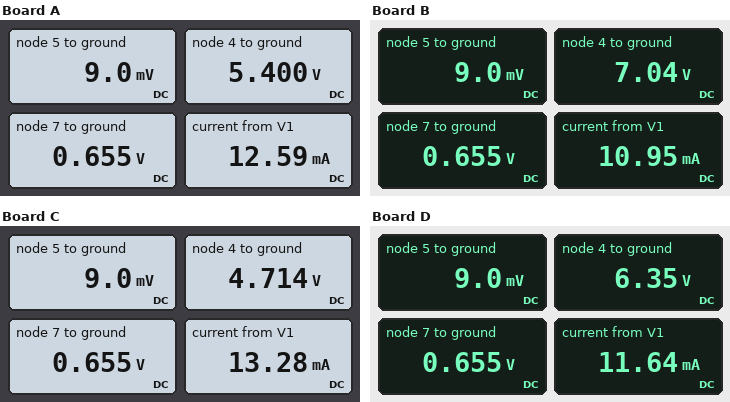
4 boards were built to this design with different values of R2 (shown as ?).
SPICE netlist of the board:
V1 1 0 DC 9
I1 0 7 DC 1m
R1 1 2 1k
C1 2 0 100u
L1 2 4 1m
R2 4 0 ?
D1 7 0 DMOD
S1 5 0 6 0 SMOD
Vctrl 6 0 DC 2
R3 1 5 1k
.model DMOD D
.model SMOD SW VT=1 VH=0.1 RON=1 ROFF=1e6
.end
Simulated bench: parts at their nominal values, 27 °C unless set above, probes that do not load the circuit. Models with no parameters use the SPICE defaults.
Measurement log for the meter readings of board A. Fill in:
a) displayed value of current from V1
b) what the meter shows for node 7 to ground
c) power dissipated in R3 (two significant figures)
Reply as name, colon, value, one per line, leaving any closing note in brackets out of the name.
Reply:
displayed value of current from V1: 12.59 mA
what the meter shows for node 7 to ground: 0.655 V
power dissipated in R3: 81 mW
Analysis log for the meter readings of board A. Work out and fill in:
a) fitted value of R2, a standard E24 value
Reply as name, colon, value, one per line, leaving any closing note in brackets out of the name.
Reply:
fitted value of R2, a standard E24 value: 1.5 kΩ
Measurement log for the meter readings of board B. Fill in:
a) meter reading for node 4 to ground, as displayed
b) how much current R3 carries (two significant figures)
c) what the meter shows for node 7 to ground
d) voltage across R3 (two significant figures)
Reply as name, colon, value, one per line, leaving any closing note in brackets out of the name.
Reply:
meter reading for node 4 to ground, as displayed: 7.04 V
how much current R3 carries: 9.0 mA
what the meter shows for node 7 to ground: 0.655 V
voltage across R3: 9.0 V
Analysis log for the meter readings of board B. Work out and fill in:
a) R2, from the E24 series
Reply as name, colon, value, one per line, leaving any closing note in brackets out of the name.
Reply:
R2, from the E24 series: 3.6 kΩ
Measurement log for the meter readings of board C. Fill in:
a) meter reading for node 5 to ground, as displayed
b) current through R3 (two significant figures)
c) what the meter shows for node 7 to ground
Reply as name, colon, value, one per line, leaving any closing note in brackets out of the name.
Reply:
meter reading for node 5 to ground, as displayed: 9.0 mV
current through R3: 9.0 mA
what the meter shows for node 7 to ground: 0.655 V
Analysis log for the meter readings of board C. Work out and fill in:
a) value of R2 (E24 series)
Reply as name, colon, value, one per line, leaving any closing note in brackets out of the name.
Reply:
value of R2: 1.1 kΩ
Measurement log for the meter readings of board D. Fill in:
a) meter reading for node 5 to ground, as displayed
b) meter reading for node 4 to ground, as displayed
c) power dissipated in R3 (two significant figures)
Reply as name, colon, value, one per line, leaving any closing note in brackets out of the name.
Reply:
meter reading for node 5 to ground, as displayed: 9.0 mV
meter reading for node 4 to ground, as displayed: 6.35 V
power dissipated in R3: 81 mW
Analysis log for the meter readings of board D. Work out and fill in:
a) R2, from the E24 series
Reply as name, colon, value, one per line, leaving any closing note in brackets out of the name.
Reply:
R2, from the E24 series: 2.4 kΩ
